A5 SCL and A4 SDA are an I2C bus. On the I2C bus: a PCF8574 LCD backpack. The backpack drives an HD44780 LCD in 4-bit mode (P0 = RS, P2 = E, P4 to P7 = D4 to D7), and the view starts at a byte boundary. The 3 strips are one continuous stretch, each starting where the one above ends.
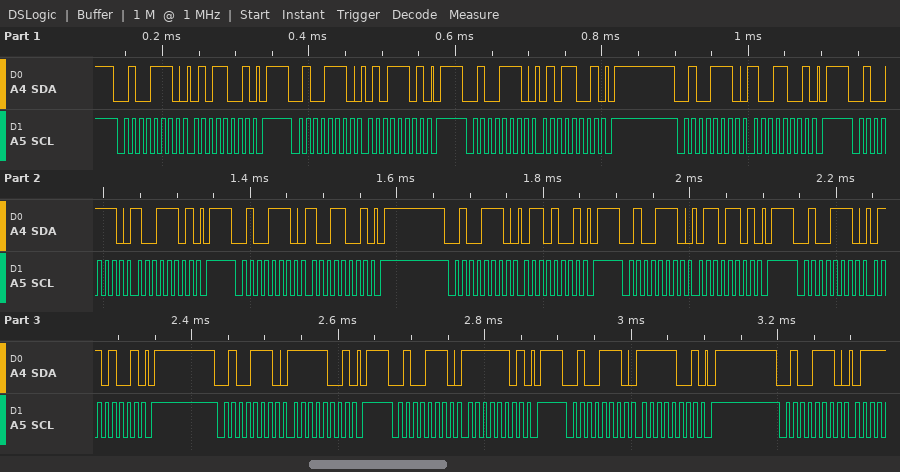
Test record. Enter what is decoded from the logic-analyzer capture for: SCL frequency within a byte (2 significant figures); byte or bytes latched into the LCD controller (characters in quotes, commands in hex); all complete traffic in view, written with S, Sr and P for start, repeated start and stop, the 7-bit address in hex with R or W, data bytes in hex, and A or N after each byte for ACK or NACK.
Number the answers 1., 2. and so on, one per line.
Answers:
1. 100 kHz
2. 'Y' 'o'
3. S 27W A 59 A P S 27W A 5D A P S 27W A 59 A P S 27W A 99 A P S 27W A 9D A P S 27W A 99 A P S 27W A 69 A P S 27W A 6D A P S 27W A 69 A P S 27W A F9 A P S 27W A FD A P S 27W A F9 A P S 27W A
